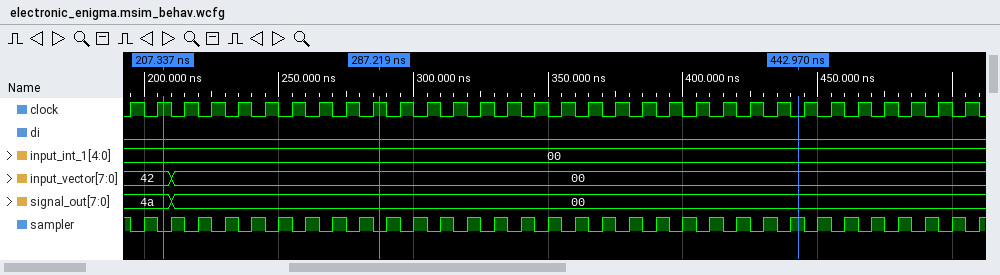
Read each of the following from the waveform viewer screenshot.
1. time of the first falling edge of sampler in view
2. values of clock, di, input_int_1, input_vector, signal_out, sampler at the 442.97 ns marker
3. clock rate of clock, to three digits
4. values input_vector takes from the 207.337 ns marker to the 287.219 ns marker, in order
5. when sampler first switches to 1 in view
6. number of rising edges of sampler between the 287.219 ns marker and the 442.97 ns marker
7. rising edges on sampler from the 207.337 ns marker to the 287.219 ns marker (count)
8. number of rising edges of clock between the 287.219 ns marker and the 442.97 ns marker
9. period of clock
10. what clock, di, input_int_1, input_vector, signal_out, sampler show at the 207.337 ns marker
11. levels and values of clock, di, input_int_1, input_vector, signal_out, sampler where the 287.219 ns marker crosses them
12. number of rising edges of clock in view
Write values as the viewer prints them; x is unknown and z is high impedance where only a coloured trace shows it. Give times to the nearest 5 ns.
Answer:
195 ns
clock=0, di=0, input_int_1=00, input_vector=00, signal_out=00, sampler=1
100 MHz
42, 00
200 ns
16
8
15
10 ns
clock=1, di=0, input_int_1=00, input_vector=42, signal_out=4a, sampler=0
clock=1, di=0, input_int_1=00, input_vector=00, signal_out=00, sampler=0
32
